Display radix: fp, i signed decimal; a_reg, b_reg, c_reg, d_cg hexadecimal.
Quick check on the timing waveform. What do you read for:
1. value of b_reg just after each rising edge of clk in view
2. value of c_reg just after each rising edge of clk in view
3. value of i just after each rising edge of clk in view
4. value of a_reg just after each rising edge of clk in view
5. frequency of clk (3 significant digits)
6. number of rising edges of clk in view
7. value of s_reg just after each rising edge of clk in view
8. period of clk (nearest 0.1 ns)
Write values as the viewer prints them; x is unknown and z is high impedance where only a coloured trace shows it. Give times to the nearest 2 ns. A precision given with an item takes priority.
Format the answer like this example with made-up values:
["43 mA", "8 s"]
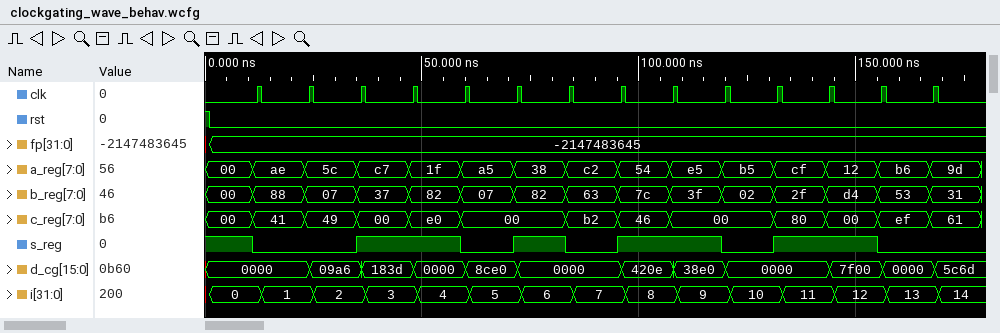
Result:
["88, 07, 37, 82, 07, 82, 63, 7c, 3f, 02, 2f, d4, 53, 31", "41, 49, 00, e0, 00, 00, b2, 46, 00, 00, 80, 00, ef, 61", "0, 1, 2, 3, 4, 5, 6, 7, 8, 9, 10, 11, 12, 13", "ae, 5c, c7, 1f, a5, 38, c2, 54, e5, b5, cf, 12, b6, 9d", "83.3 MHz", "14", "0 0 1 1 0 1 0 1 1 0 1 1 0 0", "12 ns"]
